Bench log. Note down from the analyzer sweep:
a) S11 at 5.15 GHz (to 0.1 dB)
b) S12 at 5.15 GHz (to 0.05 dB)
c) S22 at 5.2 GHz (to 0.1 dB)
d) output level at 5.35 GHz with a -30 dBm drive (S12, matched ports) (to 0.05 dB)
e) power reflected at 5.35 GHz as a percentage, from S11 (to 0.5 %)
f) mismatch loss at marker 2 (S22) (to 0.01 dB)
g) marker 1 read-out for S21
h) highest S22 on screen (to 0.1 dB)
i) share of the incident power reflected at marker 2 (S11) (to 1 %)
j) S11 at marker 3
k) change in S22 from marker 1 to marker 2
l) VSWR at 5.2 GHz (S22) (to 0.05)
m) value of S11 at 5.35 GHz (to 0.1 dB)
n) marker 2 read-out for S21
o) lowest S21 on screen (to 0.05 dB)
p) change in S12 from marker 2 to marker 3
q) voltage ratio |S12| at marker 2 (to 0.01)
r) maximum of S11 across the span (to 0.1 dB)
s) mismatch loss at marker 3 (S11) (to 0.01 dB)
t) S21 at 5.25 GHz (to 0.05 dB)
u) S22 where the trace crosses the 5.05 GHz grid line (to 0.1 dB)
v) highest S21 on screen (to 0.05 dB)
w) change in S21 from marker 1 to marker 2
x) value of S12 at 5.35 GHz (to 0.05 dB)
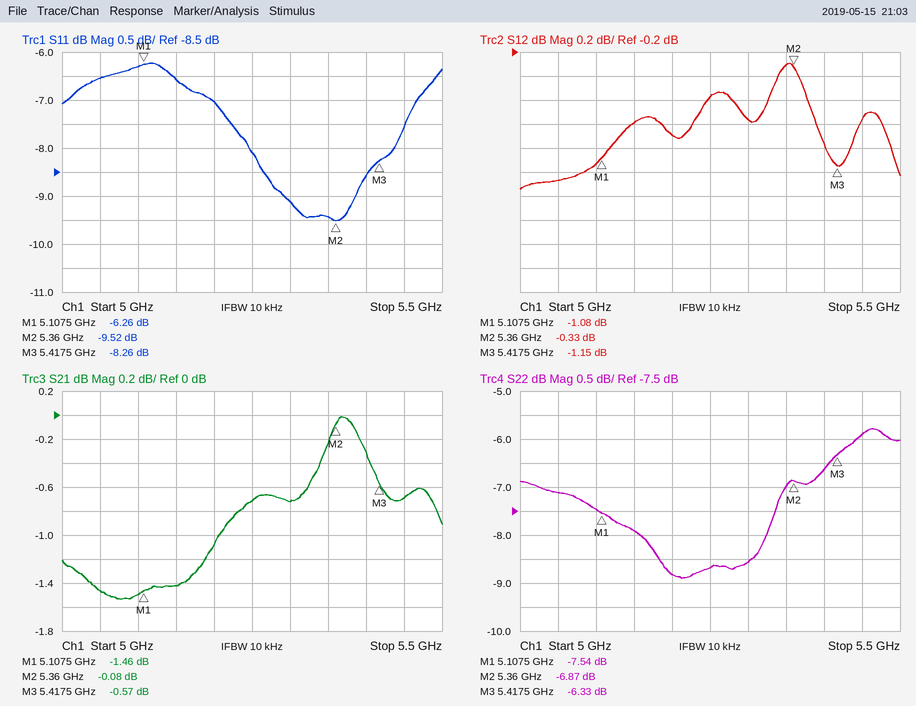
-6.6 dB
-0.80 dB
-8.8 dB
-30.30 dBm
11.5 %
1.00 dB
-1.46 dB
-5.8 dB
11 %
-8.26 dB
0.67 dB
2.15
-9.4 dB
-0.08 dB
-1.55 dB
-0.82 dB
0.96
-6.2 dB
0.70 dB
-0.70 dB
-7.1 dB
0.00 dB
1.38 dB
-0.30 dB
